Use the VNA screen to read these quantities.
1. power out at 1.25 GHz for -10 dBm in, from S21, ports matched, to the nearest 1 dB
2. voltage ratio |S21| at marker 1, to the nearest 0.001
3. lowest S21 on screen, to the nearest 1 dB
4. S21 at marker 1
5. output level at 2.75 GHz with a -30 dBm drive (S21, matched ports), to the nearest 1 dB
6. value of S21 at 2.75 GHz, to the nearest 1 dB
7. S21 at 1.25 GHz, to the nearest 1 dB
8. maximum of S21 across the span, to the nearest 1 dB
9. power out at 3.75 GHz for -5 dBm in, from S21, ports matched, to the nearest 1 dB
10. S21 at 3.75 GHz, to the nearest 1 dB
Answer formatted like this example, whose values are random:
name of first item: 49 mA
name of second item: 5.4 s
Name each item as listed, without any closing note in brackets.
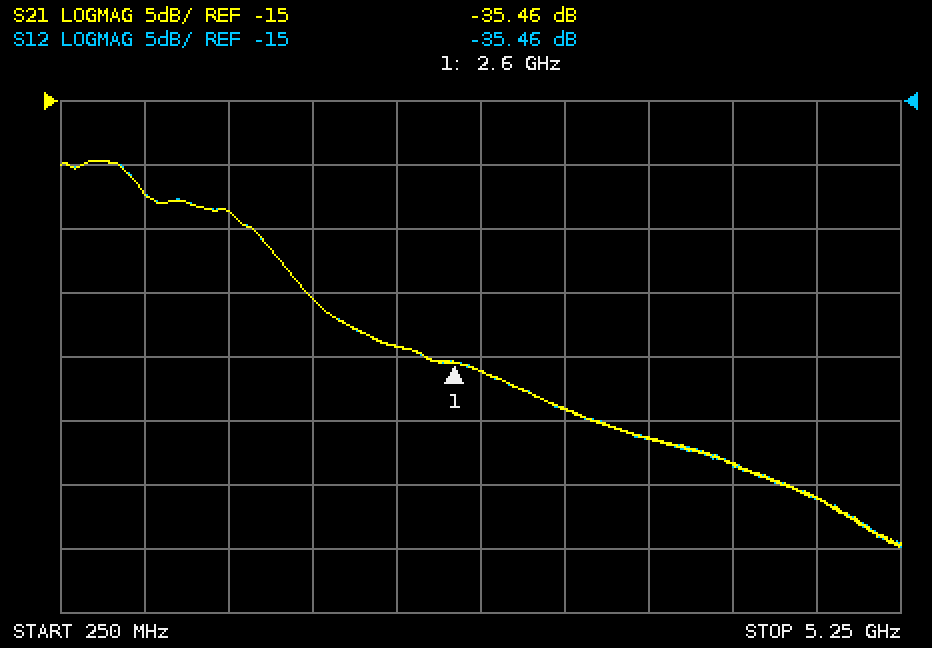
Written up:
power out at 1.25 GHz for -10 dBm in, from S21, ports matched, to the nearest 1 dB: -34 dBm
voltage ratio |S21| at marker 1, to the nearest 0.001: 0.017
lowest S21 on screen, to the nearest 1 dB: -50 dB
S21 at marker 1: -35.46 dB
output level at 2.75 GHz with a -30 dBm drive (S21, matched ports), to the nearest 1 dB: -66 dBm
value of S21 at 2.75 GHz, to the nearest 1 dB: -36 dB
S21 at 1.25 GHz, to the nearest 1 dB: -24 dB
maximum of S21 across the span, to the nearest 1 dB: -20 dB
power out at 3.75 GHz for -5 dBm in, from S21, ports matched, to the nearest 1 dB: -46 dBm
S21 at 3.75 GHz, to the nearest 1 dB: -41 dB
